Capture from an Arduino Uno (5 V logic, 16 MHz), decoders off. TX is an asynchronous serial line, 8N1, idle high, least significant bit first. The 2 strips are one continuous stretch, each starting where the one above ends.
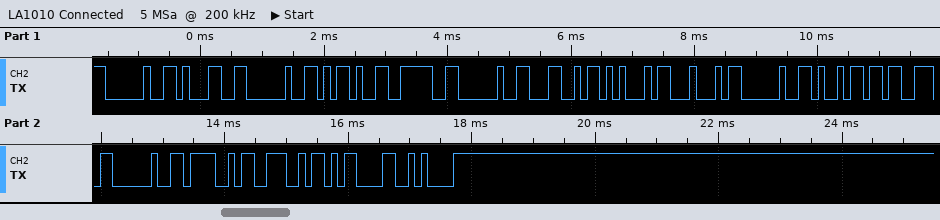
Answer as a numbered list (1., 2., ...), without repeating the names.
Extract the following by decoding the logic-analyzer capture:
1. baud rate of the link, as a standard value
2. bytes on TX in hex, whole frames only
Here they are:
1. 9600 baud
2. 20 31 20 2D 3E 20 4C 45 44 20 69 73 20 4F 4E 0D 0A
